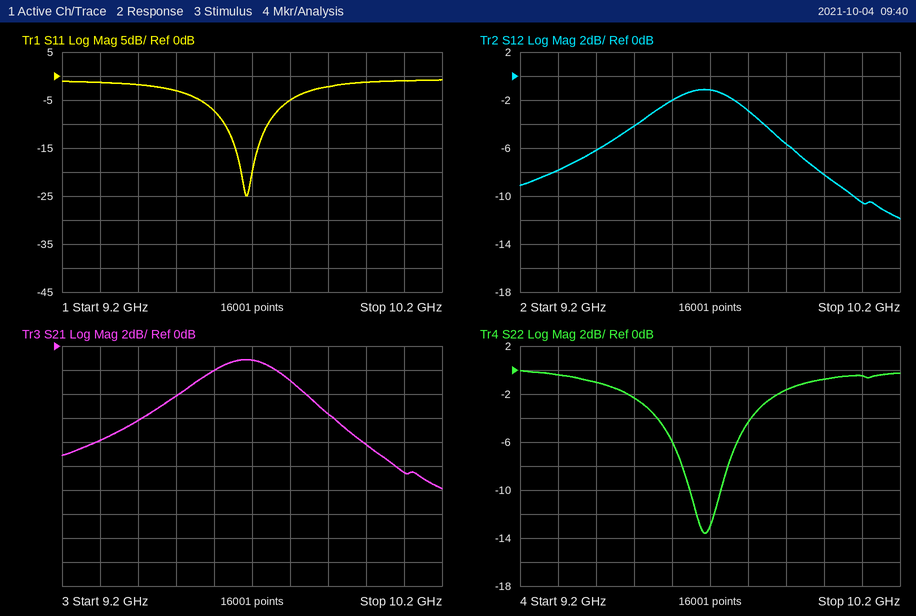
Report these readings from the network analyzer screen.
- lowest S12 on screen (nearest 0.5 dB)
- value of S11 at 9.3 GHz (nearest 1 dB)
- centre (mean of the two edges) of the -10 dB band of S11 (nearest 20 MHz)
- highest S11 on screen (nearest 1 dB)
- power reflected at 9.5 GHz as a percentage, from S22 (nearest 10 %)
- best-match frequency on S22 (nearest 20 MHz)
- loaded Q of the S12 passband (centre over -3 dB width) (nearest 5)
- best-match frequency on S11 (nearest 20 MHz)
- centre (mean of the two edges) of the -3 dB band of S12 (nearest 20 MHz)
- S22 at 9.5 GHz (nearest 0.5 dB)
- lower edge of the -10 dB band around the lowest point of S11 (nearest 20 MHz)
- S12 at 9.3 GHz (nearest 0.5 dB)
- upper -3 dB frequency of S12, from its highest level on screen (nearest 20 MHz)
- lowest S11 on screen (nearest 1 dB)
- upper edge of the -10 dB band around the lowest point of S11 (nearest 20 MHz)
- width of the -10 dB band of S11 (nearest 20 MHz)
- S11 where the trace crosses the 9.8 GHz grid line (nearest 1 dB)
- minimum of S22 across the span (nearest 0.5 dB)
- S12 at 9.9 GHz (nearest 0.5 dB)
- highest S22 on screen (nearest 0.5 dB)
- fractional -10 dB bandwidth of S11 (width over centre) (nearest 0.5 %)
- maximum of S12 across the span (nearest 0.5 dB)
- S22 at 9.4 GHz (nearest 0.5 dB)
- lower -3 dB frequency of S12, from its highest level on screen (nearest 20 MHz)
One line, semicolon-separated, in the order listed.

-12.0 dB; -1 dB; 9.68 GHz; -1 dB; 60 %; 9.68 GHz; 30; 9.68 GHz; 9.68 GHz; -2.5 dB; 9.62 GHz; -8.0 dB; 9.84 GHz; -25 dB; 9.74 GHz; 120 MHz; -5 dB; -13.5 dB; -5.5 dB; 0.0 dB; 1.0 %; -1.0 dB; -1.0 dB; 9.50 GHz
